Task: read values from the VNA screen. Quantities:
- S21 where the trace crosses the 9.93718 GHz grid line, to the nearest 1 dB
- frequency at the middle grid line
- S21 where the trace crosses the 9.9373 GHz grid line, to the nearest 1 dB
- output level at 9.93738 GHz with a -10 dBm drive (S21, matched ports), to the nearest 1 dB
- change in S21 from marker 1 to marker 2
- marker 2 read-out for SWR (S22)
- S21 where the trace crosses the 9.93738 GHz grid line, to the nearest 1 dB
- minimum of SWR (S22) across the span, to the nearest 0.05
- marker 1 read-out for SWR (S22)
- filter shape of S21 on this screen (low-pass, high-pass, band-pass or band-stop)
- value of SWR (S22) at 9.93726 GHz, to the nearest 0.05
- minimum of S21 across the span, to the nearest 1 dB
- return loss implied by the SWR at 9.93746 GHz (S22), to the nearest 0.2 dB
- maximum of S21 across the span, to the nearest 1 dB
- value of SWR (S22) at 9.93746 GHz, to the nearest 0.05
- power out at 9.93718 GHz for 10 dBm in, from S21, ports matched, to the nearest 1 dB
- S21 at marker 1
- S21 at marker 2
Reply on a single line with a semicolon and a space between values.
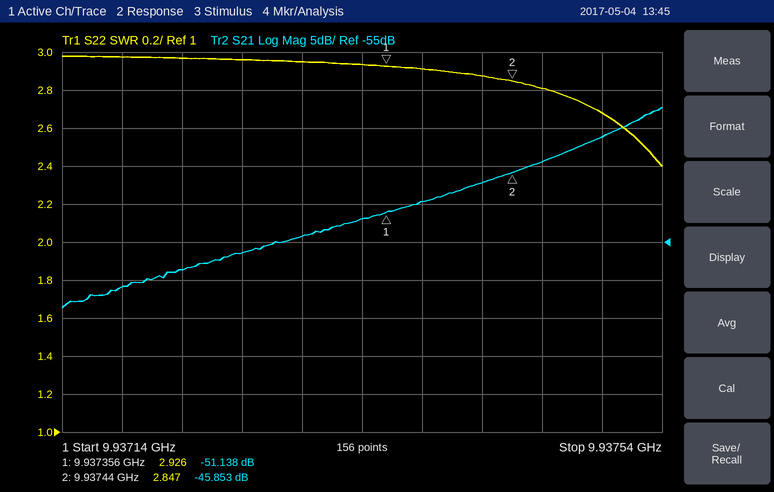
-61 dB; 9.93734 GHz; -54 dB; -60 dBm; 5.285 dB; 2.847; -50 dB; 2.40; 2.926; high-pass; 2.95; -64 dB; 6.4 dB; -37 dB; 2.80; -51 dBm; -51.138 dB; -45.853 dB
